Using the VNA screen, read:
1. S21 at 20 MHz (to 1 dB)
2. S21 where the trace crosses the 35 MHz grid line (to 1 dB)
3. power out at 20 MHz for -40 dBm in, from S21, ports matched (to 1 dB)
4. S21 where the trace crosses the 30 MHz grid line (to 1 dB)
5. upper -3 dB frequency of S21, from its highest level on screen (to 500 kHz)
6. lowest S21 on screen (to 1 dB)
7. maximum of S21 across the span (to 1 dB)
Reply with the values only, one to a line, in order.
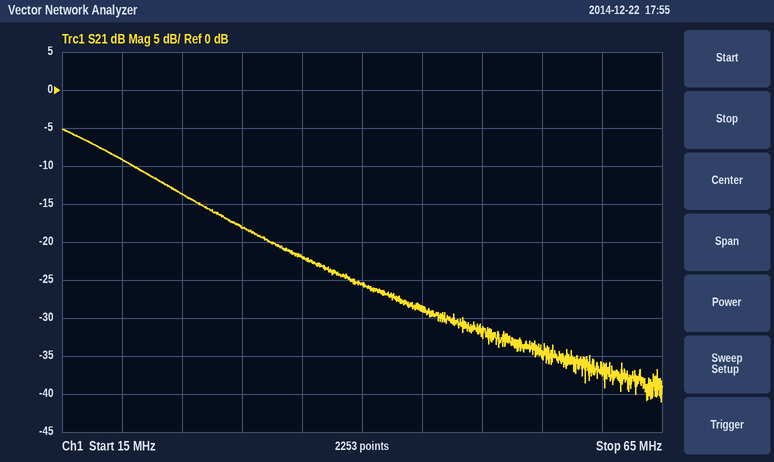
-9 dB
-22 dB
-49 dBm
-18 dB
19.0 MHz
-41 dB
-5 dB
